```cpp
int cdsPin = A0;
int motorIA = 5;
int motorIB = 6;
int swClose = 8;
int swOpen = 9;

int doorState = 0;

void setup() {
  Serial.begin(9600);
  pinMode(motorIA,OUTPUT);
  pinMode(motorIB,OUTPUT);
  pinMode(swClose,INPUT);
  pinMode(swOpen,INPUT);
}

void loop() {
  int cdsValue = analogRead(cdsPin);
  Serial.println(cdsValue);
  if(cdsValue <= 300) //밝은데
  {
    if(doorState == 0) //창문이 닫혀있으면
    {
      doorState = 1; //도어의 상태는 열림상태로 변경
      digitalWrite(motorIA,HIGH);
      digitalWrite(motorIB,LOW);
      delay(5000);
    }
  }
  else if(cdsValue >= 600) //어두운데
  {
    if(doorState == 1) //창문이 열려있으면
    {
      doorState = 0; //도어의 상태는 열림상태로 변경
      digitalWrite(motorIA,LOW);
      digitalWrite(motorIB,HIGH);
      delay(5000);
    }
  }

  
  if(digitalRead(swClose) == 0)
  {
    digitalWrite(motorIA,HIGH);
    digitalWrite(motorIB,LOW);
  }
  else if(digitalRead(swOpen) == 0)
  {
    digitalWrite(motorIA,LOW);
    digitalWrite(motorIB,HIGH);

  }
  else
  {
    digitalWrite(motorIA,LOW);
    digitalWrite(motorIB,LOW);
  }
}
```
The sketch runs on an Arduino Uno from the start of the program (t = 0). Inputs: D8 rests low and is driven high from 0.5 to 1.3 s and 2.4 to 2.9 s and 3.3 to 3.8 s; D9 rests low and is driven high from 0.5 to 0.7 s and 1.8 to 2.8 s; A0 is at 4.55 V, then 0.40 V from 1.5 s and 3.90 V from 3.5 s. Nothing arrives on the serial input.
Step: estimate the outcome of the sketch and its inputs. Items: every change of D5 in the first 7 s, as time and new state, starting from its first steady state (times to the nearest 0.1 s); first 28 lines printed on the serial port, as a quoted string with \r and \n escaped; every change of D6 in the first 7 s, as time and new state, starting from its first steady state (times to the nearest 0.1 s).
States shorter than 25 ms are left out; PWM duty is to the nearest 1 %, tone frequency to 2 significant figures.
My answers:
0 s high; 0.5 s low; 1.3 s high; 6.5 s low
"931\r\n931\r\n931\r\n931\r\n931\r\n931\r\n931\r\n931\r\n931\r\n931\r\n931\r\n931\r\n931\r\n931\r\n931\r\n931\r\n931\r\n931\r\n931\r\n931\r\n931\r\n931\r\n931\r\n931\r\n931\r\n931\r\n931\r\n931\r\n"
0 s low; 0.7 s high; 1.3 s low; 6.5 s high
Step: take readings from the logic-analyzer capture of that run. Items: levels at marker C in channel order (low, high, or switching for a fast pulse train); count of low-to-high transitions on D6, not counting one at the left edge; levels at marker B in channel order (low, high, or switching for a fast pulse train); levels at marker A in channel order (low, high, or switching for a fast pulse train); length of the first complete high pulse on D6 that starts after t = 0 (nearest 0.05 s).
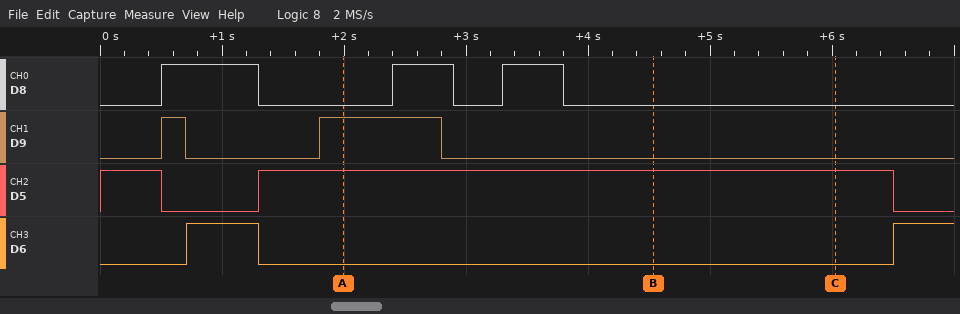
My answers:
D8 low, D9 low, D5 high, D6 low
2
D8 low, D9 low, D5 high, D6 low
D8 low, D9 high, D5 high, D6 low
0.60 s
